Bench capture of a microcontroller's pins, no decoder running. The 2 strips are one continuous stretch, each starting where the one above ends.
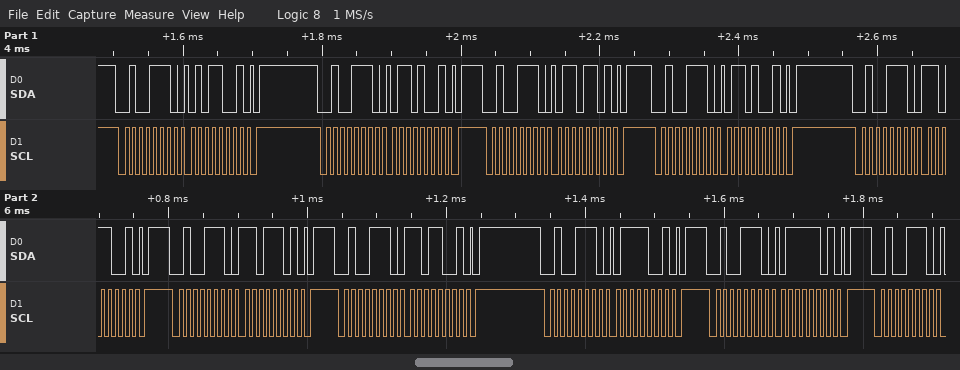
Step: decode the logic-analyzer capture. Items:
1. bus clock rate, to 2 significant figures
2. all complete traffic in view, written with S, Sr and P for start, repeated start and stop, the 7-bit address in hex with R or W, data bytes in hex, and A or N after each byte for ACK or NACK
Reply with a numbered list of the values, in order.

1. 100 kHz
2. S 27W A 59 A P S 27W A 69 A P S 27W A 6D A P S 27W A 69 A P S 27W A D9 A P S 27W A DD A P S 27W A D9 A P S 27W A 79 A P S 27W A 7D A P S 27W A
